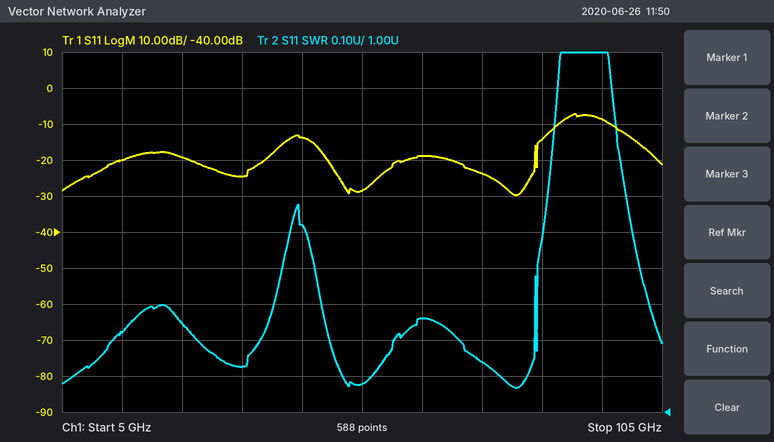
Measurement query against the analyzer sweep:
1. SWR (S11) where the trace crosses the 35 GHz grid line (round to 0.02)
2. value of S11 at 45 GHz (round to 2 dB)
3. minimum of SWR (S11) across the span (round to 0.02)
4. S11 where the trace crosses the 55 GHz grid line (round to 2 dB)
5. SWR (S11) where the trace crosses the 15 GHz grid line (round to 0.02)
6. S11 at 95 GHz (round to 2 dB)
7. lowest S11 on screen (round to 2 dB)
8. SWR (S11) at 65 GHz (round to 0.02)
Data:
1.12
-14 dB
1.06
-28 dB
1.22
-8 dB
-30 dB
1.26
